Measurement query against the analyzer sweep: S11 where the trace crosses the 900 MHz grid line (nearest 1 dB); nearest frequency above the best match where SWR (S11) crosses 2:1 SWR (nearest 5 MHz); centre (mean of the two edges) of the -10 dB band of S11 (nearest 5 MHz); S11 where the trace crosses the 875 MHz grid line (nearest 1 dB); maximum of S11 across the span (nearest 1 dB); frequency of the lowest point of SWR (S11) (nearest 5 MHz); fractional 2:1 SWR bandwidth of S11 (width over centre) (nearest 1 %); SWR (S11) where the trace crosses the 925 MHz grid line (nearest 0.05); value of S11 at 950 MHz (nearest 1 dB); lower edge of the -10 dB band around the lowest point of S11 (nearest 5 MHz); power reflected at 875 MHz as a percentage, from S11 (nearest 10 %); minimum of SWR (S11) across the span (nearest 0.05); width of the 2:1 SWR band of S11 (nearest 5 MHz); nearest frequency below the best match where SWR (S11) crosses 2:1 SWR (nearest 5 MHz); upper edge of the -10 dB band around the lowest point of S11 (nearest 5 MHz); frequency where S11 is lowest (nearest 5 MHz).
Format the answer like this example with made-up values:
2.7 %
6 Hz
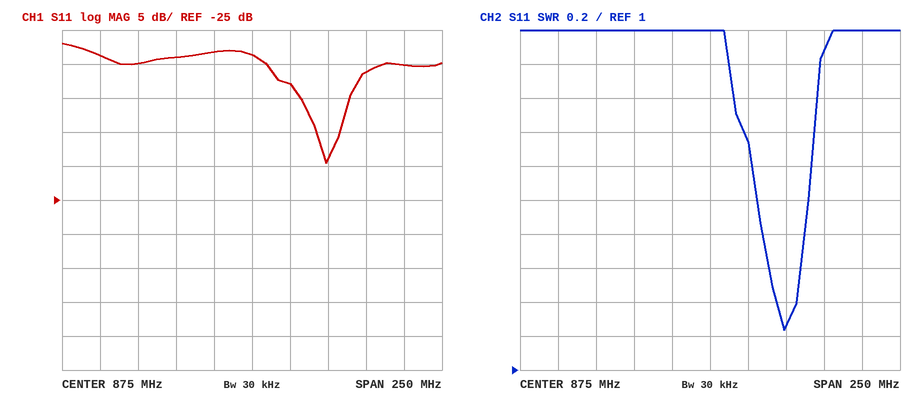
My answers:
-8 dB
940 MHz
925 MHz
-4 dB
-2 dB
925 MHz
4 %
1.25
-6 dB
905 MHz
40 %
1.25
35 MHz
905 MHz
940 MHz
925 MHz
